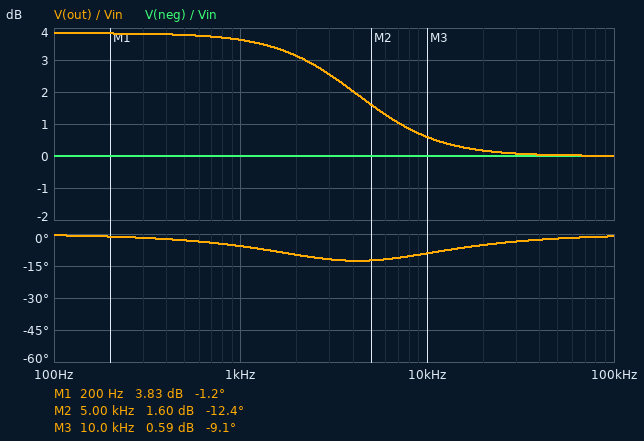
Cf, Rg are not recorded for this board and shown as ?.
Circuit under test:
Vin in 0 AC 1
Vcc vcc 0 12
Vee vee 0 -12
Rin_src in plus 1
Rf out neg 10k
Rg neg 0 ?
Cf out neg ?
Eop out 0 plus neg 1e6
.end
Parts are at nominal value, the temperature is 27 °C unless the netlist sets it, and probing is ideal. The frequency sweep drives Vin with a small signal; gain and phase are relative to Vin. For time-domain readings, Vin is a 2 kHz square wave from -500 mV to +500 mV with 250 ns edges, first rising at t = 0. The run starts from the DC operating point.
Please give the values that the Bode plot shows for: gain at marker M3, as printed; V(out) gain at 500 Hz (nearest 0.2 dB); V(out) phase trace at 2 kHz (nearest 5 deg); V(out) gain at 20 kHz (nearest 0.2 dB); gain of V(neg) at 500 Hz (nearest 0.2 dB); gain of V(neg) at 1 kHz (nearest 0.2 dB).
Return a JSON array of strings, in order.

["0.59 dB", "3.8 dB", "-10 deg", "0.2 dB", "0 dB", "0 dB"]
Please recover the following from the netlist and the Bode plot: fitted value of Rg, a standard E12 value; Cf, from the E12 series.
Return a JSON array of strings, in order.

["18 kΩ", "4.7 nF"]
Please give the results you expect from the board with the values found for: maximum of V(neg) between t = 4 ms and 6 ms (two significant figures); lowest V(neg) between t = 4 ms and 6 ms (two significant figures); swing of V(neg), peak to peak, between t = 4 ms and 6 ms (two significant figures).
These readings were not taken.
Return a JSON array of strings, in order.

["500 mV", "-500 mV", "1.0 V"]
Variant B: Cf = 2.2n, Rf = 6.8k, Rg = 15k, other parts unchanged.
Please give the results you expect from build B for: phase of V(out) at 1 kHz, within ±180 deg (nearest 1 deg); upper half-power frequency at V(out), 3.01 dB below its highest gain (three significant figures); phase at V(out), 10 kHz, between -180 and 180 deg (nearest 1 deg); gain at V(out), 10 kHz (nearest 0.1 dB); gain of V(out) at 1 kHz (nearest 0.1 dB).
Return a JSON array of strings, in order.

["-2 deg", "46.2 kHz", "-10 deg", "2.0 dB", "3.2 dB"]
